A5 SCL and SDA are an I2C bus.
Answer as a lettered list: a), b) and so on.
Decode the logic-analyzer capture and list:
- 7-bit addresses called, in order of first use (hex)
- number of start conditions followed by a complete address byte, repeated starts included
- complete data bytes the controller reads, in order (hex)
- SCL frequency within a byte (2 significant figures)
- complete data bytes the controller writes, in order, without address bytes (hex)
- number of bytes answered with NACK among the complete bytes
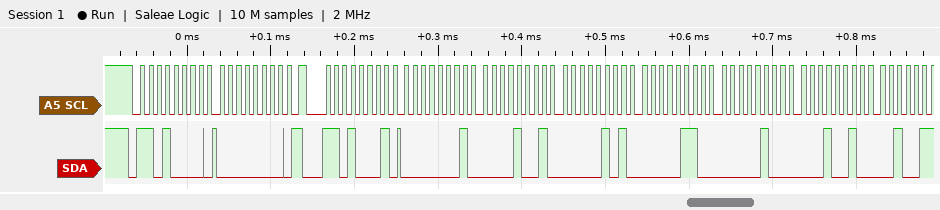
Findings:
a) 0x68
b) 2
c) 01 09 05 06 04 12
d) 100 kHz
e) 00
f) 0
